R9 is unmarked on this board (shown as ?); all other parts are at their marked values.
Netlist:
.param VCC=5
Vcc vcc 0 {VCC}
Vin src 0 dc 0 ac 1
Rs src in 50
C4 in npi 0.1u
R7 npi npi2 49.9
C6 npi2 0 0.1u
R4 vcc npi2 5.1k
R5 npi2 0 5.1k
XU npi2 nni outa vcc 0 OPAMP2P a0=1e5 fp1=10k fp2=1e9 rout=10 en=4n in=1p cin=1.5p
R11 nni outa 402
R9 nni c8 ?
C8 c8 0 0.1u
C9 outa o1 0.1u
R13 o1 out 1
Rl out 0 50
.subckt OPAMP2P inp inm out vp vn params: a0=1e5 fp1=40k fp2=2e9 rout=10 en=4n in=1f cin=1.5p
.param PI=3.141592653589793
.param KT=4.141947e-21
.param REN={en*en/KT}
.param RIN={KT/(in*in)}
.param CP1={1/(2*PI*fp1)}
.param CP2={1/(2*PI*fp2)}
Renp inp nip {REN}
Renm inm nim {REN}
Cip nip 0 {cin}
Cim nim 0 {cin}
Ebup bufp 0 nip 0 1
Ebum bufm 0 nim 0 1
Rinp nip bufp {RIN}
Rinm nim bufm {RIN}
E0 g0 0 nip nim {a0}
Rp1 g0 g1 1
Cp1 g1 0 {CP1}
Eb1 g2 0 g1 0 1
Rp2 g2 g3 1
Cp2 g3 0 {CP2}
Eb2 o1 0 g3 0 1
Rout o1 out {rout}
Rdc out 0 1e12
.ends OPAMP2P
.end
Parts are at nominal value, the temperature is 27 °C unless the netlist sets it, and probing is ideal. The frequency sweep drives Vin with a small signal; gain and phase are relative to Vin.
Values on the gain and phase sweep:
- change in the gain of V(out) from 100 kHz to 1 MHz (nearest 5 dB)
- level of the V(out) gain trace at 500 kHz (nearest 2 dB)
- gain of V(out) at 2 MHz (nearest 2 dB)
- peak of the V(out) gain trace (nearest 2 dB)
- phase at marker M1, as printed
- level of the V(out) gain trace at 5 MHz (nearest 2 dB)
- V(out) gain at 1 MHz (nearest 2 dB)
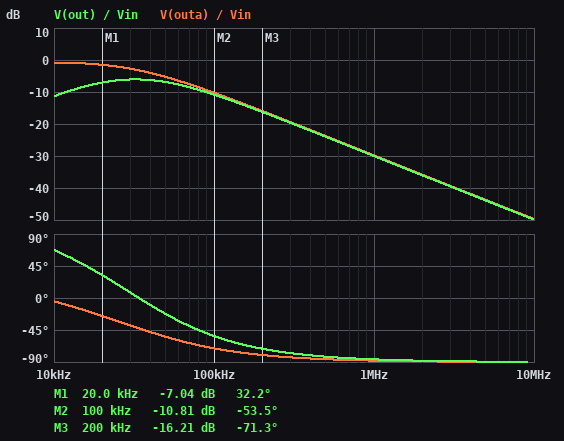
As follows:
-20 dB
-24 dB
-36 dB
-6 dB
32.2 deg
-44 dB
-30 dB
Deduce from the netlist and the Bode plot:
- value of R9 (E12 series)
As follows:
390 Ω
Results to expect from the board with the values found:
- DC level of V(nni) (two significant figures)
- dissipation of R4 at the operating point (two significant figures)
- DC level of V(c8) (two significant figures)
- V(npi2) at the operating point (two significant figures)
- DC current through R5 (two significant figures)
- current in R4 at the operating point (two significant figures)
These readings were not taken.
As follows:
2.5 V
1.2 mW
2.5 V
2.5 V
490 µA
490 µA
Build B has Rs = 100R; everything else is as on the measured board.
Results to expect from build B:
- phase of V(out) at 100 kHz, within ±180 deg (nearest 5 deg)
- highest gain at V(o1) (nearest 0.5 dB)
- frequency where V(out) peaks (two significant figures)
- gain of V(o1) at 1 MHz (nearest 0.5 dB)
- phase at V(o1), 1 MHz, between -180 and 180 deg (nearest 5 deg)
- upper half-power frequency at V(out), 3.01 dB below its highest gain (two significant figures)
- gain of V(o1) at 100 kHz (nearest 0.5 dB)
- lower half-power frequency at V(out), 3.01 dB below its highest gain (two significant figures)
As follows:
-60 deg
-8.0 dB
26 kHz
-33.5 dB
-85 deg
64 kHz
-14.0 dB
11 kHz
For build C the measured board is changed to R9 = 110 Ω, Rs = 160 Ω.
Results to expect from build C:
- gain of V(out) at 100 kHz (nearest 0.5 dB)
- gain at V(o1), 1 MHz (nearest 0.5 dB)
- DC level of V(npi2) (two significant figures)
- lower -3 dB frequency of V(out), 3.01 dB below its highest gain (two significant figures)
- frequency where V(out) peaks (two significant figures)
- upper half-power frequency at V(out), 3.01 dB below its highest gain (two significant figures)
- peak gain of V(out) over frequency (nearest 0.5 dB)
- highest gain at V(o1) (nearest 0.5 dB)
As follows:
-10.0 dB
-29.0 dB
2.5 V
13 kHz
28 kHz
65 kHz
-4.0 dB
-3.5 dB
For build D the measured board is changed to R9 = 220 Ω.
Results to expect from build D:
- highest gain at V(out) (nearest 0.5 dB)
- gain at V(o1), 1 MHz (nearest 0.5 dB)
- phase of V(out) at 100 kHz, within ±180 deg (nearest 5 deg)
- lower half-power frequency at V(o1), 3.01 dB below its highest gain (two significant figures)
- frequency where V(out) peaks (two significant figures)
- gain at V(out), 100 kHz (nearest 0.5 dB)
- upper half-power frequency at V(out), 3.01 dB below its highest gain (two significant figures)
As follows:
-3.5 dB
-27.0 dB
-50 deg
15 kHz
33 kHz
-8.0 dB
78 kHz
